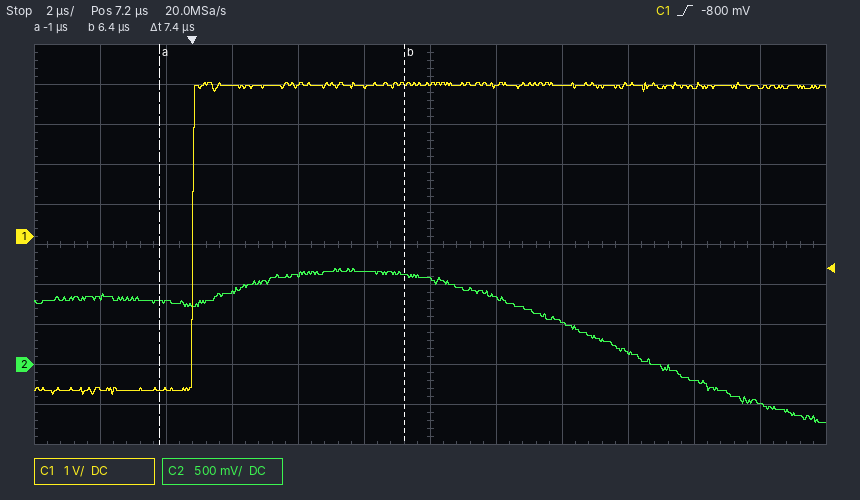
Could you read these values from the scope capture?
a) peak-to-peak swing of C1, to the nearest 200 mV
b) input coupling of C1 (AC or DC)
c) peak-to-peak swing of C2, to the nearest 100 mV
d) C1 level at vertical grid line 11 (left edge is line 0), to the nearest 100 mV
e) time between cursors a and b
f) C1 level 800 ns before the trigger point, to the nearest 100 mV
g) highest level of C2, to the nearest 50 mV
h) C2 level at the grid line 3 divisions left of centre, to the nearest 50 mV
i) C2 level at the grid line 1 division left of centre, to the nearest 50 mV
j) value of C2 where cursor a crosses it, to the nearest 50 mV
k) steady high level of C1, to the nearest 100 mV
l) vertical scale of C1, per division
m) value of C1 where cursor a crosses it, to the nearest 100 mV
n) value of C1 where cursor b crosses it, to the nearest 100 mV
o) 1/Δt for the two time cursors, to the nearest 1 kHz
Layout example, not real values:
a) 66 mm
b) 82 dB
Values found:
a) 7.8 V
b) DC
c) 1.90 V
d) 3.7 V
e) 7.4 µs
f) -3.8 V
g) 1.20 V
h) 900 mV
i) 1.15 V
j) 800 mV
k) 3.8 V
l) 1 V
m) -3.8 V
n) 3.8 V
o) 135 kHz
